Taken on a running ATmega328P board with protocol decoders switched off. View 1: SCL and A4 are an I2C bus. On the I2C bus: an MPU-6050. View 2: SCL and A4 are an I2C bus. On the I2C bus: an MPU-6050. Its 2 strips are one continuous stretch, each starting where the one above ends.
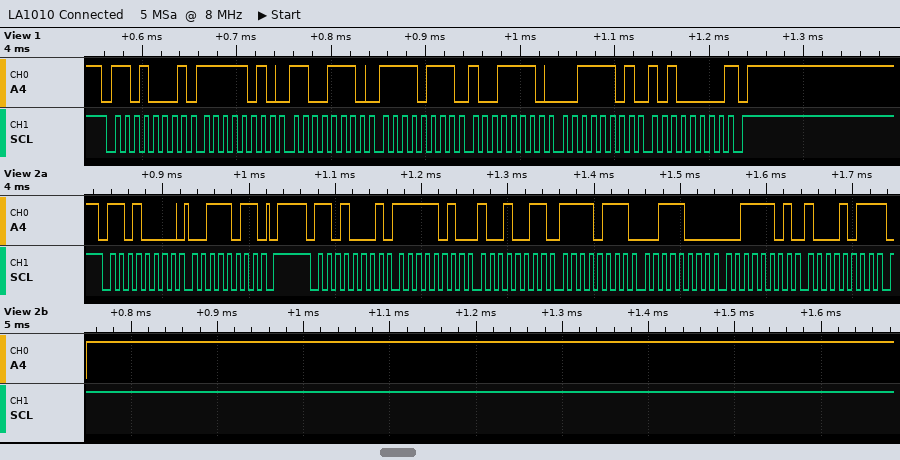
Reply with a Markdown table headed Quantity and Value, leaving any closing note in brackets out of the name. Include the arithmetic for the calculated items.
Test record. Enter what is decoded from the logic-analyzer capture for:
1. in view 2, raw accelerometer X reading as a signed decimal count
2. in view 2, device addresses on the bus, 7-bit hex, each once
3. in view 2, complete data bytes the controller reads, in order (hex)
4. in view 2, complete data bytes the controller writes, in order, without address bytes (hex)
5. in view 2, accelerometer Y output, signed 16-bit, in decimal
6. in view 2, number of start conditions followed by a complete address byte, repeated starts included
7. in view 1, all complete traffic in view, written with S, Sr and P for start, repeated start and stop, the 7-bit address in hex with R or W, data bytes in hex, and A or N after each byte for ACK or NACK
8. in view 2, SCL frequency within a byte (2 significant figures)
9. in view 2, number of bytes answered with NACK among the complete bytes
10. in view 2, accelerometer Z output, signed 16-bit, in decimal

| Quantity | Value |
|---|---|
| in view 2, raw accelerometer X reading as a signed decimal count | 0xFA93 = -1389 |
| in view 2, device addresses on the bus, 7-bit hex, each once | 0x68 |
| in view 2, complete data bytes the controller reads, in order | FA 93 F7 38 3D 8B |
| in view 2, complete data bytes the controller writes, in order, without address bytes | 3B |
| in view 2, accelerometer Y output, signed 16-bit, in decimal | 0xF738 = -2248 |
| in view 2, number of start conditions followed by a complete address byte, repeated starts included | 2 |
| in view 1, all complete traffic in view, written with S, Sr and P for start, repeated start and stop, the 7-bit address in hex with R or W, data bytes in hex, and A or N after each byte for ACK or NACK | S 68R A FA A CE A F7 A 9E A 3D A A0 N P |
| in view 2, SCL frequency within a byte | 100 kHz |
| in view 2, number of bytes answered with NACK among the complete bytes | 1 |
| in view 2, accelerometer Z output, signed 16-bit, in decimal | 0x3D8B = 15755 |
